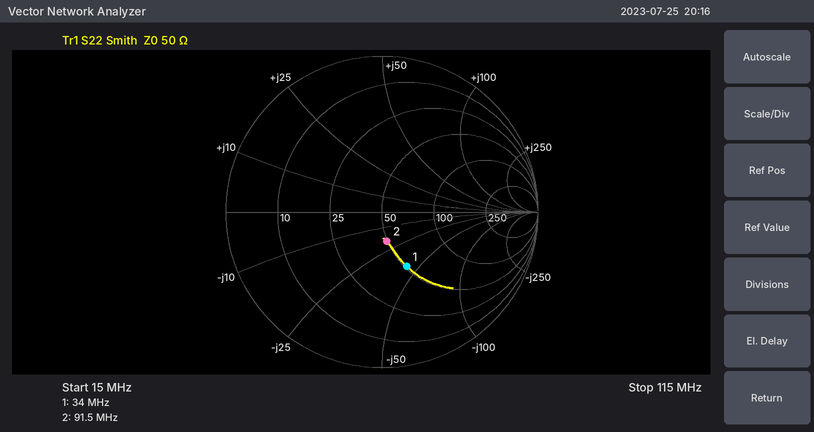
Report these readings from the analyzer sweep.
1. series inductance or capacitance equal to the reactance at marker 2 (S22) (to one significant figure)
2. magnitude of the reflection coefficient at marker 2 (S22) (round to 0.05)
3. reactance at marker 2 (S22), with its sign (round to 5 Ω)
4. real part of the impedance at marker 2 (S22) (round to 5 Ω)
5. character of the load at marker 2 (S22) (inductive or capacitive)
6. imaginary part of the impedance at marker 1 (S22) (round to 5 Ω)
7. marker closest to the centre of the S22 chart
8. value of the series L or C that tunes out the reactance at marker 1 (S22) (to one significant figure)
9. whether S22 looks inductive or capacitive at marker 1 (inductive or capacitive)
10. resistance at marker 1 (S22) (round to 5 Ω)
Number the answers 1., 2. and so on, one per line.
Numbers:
1. 90 pF
2. 0.20
3. -20 Ω
4. 50 Ω
5. capacitive
6. -40 Ω
7. marker 2
8. 200 nH
9. capacitive
10. 50 Ω
